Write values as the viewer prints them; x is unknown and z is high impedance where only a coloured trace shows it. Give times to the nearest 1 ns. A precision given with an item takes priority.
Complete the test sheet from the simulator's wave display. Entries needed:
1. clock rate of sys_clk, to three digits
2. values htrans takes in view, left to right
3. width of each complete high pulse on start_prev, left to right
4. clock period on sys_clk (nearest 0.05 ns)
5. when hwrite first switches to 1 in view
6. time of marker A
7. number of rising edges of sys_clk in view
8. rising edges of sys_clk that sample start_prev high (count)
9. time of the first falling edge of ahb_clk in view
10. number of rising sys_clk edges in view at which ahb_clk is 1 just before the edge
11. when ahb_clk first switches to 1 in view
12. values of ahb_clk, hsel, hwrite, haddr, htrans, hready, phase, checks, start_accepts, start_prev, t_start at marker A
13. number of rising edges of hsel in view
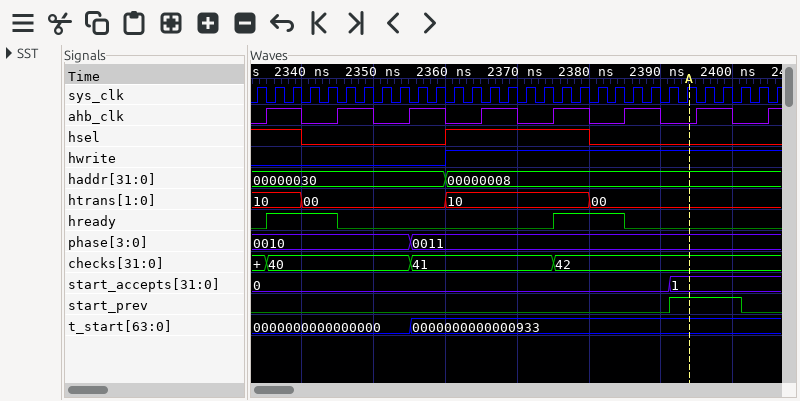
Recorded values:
400 MHz
10, 00, 10, 00
10 ns
2.5 ns
2360 ns
2394 ns
30
4
2340 ns
15
2335 ns
ahb_clk=0, hsel=0, hwrite=1, haddr=00000008, htrans=00, hready=0, phase=0011, checks=42, start_accepts=1, start_prev=1, t_start=0000000000000933
1
